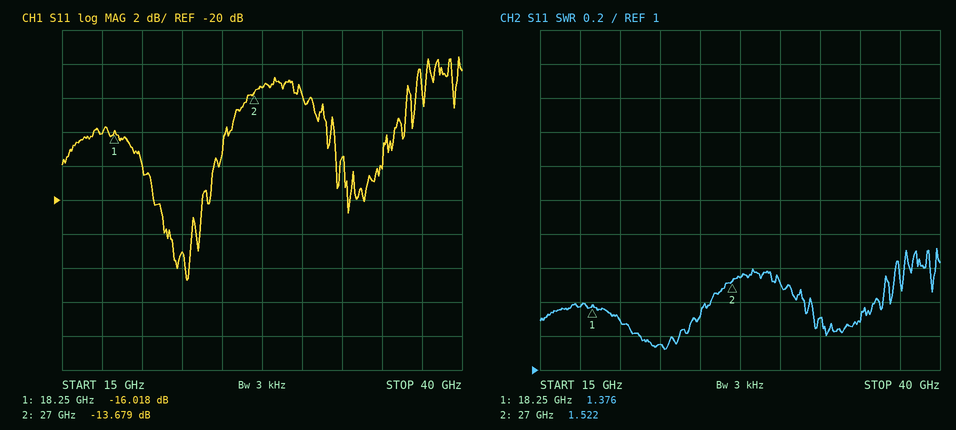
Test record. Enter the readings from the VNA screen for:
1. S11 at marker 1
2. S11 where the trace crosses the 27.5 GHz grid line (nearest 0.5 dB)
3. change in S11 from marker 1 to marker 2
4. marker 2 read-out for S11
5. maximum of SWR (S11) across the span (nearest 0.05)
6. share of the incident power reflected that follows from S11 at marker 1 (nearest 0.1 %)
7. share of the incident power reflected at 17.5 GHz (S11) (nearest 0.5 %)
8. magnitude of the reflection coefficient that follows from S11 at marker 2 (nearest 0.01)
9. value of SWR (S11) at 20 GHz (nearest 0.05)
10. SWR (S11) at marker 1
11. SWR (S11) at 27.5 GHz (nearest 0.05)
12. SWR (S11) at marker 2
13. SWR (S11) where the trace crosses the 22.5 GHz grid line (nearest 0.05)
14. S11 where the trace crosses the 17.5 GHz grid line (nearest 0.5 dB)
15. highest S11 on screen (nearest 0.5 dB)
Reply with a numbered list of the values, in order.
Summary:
1. -16.018 dB
2. -13.5 dB
3. 2.339 dB
4. -13.679 dB
5. 1.70
6. 2.5 %
7. 2.5 %
8. 0.21
9. 1.30
10. 1.376
11. 1.55
12. 1.522
13. 1.15
14. -16.0 dB
15. -11.5 dB
